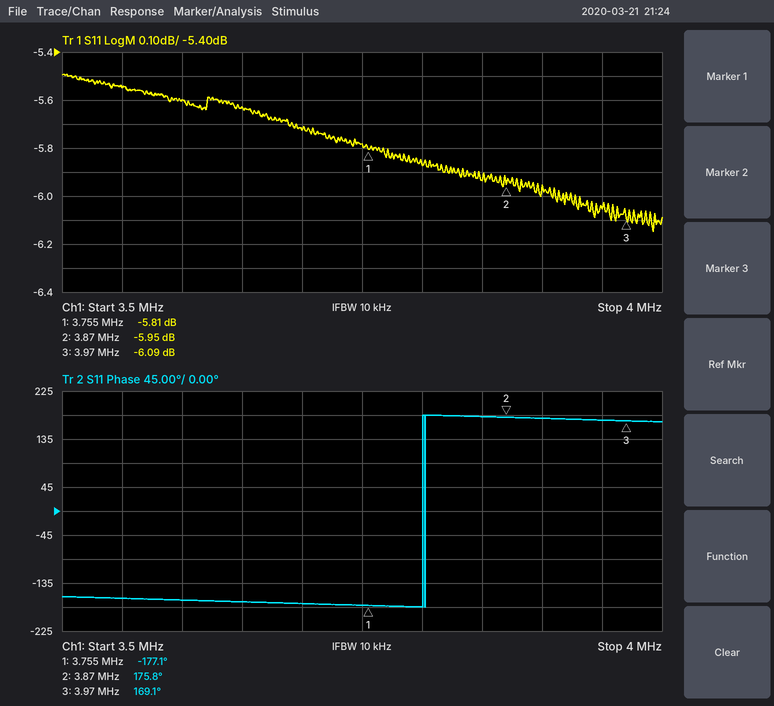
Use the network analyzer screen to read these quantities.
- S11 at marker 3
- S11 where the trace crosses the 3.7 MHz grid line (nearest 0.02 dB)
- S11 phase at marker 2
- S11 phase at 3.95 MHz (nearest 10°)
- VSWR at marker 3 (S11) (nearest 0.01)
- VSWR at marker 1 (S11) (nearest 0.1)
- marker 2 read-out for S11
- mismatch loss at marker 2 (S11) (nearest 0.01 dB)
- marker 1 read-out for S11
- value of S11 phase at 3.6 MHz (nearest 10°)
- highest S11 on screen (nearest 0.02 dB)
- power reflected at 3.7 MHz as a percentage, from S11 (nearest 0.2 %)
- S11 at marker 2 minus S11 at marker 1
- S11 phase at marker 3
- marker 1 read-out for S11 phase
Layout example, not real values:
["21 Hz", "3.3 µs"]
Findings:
["-6.09 dB", "-5.72 dB", "175.8°", "170°", "2.97", "3.1", "-5.95 dB", "1.27 dB", "-5.81 dB", "-170°", "-5.50 dB", "26.8 %", "-0.14 dB", "169.1°", "-177.1°"]
